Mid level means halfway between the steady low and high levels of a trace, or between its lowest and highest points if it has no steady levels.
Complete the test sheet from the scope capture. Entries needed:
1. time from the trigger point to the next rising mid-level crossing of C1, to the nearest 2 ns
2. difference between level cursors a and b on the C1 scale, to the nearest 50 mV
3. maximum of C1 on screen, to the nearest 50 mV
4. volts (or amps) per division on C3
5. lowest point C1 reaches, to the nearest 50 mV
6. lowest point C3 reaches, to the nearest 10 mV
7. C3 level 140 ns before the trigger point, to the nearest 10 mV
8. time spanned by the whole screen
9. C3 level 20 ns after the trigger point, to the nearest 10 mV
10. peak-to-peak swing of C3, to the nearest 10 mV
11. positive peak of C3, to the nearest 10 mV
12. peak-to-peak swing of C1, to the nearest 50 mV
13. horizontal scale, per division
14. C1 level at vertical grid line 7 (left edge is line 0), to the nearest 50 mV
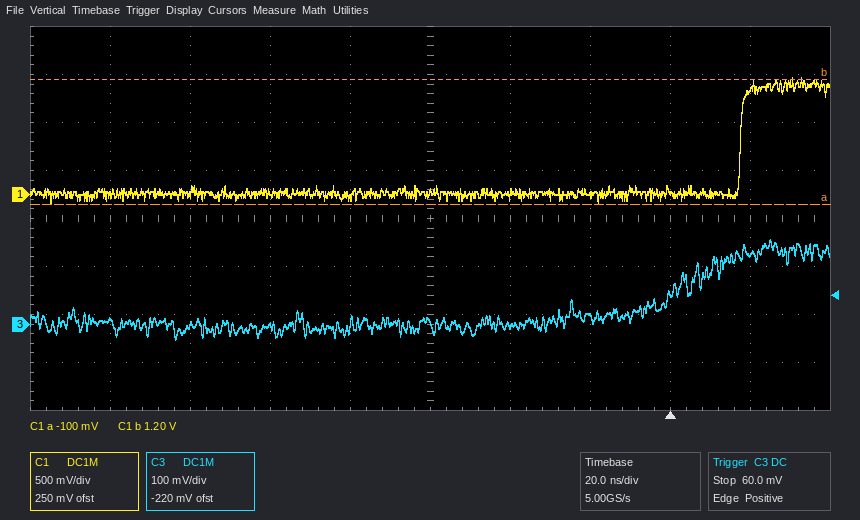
18 ns
1.30 V
1.20 V
100 mV
-100 mV
-30 mV
0 mV
200 ns
150 mV
210 mV
180 mV
1.30 V
20 ns
0 mV
